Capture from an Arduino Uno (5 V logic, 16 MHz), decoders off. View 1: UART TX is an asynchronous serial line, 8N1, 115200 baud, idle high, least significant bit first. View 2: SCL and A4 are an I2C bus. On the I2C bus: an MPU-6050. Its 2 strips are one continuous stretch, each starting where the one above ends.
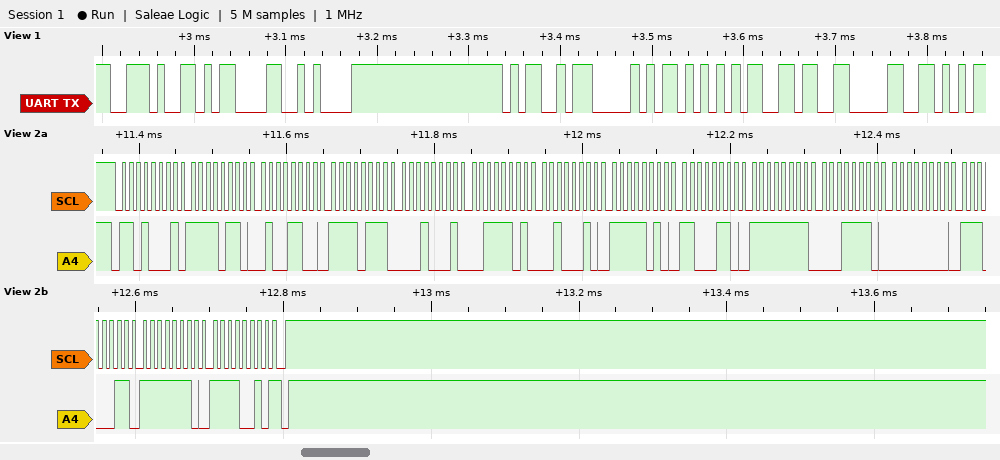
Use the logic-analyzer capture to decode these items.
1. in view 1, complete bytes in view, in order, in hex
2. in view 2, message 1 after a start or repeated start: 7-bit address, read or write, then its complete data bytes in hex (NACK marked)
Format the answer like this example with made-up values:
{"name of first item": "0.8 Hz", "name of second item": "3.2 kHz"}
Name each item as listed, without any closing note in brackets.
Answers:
{"in view 1, complete bytes in view, in order, in hex": "0x2E 0x0D 0x0A 0x4D 0x50 0x55 0x36 0x30", "in view 2, message 1 after a start or repeated start: 7-bit address, read or write, then its complete data bytes in hex": "0x68 read: F6 4C F7 11 3D 22 FA C6 FF 1E 00 E3 FE F2 NACK"}
